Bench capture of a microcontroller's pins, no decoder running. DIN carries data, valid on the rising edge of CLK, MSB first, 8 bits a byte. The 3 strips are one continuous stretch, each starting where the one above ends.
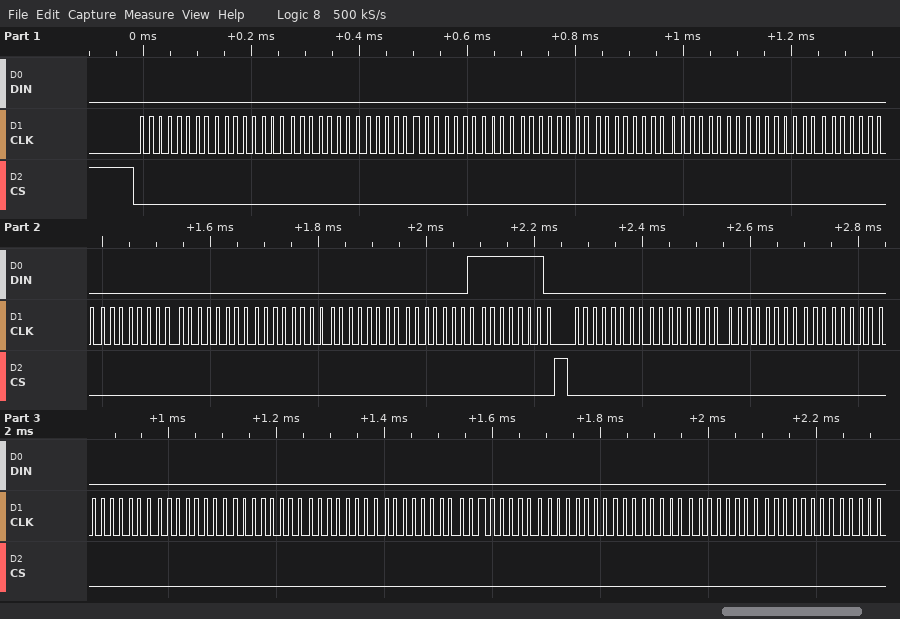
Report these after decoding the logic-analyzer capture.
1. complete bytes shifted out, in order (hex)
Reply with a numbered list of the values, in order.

1. 00 00 00 00 00 00 00 00 00 00 00 00 00 00 01 FE 00 00 00 00 00 00 00 00 00 00 00 00 00 00
